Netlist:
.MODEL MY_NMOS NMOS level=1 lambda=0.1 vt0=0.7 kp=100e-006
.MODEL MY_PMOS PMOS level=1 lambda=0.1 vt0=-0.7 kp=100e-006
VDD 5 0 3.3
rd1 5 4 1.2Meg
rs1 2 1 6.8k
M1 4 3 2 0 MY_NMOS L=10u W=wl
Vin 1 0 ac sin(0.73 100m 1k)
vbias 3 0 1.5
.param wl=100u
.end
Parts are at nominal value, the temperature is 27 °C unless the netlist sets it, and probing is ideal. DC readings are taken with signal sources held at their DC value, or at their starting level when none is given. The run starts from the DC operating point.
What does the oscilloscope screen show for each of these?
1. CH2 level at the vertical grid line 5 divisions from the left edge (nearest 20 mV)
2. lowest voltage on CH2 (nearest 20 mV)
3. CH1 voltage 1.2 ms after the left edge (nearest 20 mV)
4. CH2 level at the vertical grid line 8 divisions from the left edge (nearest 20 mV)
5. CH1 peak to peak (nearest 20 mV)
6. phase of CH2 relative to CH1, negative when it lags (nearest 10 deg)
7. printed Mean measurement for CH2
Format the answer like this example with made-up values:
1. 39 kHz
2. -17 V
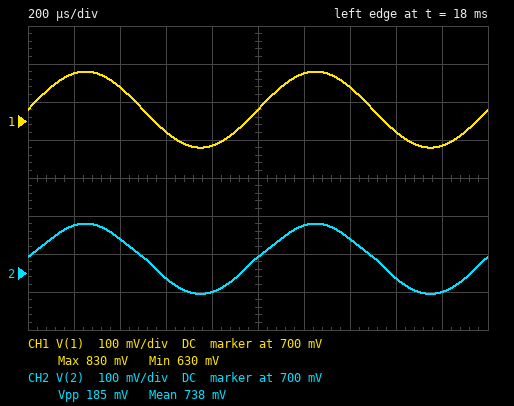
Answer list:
1. 740 mV
2. 640 mV
3. 820 mV
4. 680 mV
5. 200 mV
6. 0 deg
7. 738 mV
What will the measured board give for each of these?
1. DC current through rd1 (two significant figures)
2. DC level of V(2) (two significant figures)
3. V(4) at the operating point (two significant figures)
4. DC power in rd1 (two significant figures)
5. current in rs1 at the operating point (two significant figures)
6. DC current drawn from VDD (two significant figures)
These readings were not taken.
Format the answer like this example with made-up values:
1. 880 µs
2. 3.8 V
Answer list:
1. 1.8 µA
2. 740 mV
3. 1.2 V
4. 3.7 µW
5. 1.8 µA
6. 1.8 µA
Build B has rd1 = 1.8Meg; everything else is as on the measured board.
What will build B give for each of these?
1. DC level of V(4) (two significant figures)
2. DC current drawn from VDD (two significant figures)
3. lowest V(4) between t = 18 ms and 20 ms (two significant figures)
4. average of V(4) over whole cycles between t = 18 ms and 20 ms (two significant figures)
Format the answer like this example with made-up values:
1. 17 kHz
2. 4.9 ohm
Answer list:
1. 770 mV
2. 1.4 µA
3. 650 mV
4. 1.7 V
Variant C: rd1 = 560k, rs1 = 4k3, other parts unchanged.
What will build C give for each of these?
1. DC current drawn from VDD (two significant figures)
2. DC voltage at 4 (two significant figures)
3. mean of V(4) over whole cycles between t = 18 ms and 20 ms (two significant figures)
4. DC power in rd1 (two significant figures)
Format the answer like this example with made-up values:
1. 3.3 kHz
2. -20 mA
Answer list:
1. 2.1 µA
2. 2.1 V
3. 2.0 V
4. 2.5 µW
